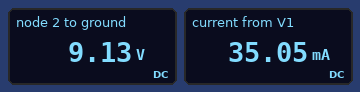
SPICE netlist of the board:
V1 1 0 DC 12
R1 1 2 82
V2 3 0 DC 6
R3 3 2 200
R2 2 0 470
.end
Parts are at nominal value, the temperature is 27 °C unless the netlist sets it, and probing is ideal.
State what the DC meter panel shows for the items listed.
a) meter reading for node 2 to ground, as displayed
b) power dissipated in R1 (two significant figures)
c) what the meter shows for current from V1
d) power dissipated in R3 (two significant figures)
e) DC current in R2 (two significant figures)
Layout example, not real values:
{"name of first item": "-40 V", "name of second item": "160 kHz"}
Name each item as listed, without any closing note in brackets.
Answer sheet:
{"meter reading for node 2 to ground, as displayed": "9.13 V", "power dissipated in R1": "100 mW", "what the meter shows for current from V1": "35.05 mA", "power dissipated in R3": "49 mW", "DC current in R2": "19 mA"}
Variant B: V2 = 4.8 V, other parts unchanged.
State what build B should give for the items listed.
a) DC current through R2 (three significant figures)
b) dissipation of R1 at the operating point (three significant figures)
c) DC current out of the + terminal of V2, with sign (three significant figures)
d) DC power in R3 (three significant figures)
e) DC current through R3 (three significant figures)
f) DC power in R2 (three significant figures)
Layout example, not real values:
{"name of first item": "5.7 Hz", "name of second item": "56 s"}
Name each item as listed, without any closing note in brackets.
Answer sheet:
{"DC current through R2": "18.8 mA", "dissipation of R1 at the operating point": "124 mW", "DC current out of the + terminal of V2, with sign": "-20.1 mA", "DC power in R3": "80.6 mW", "DC current through R3": "20.1 mA", "DC power in R2": "165 mW"}
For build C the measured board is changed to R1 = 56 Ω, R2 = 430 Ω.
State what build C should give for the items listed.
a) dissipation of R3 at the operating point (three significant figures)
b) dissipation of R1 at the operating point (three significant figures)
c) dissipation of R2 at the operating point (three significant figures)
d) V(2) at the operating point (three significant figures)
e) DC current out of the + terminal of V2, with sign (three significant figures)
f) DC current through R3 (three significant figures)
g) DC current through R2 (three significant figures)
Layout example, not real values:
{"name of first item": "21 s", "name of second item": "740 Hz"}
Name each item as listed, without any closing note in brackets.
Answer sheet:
{"dissipation of R3 at the operating point": "68.5 mW", "dissipation of R1 at the operating point": "94.4 mW", "dissipation of R2 at the operating point": "219 mW", "V(2) at the operating point": "9.70 V", "DC current out of the + terminal of V2, with sign": "-18.5 mA", "DC current through R3": "18.5 mA", "DC current through R2": "22.6 mA"}
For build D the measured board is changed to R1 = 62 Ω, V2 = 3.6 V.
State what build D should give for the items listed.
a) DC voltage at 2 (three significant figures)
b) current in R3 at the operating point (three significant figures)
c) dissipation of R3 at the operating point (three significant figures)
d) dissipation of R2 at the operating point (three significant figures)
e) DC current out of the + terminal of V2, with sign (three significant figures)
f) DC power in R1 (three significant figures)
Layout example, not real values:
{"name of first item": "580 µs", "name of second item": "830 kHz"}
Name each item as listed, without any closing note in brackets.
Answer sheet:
{"DC voltage at 2": "9.10 V", "current in R3 at the operating point": "27.5 mA", "dissipation of R3 at the operating point": "151 mW", "dissipation of R2 at the operating point": "176 mW", "DC current out of the + terminal of V2, with sign": "-27.5 mA", "DC power in R1": "136 mW"}
